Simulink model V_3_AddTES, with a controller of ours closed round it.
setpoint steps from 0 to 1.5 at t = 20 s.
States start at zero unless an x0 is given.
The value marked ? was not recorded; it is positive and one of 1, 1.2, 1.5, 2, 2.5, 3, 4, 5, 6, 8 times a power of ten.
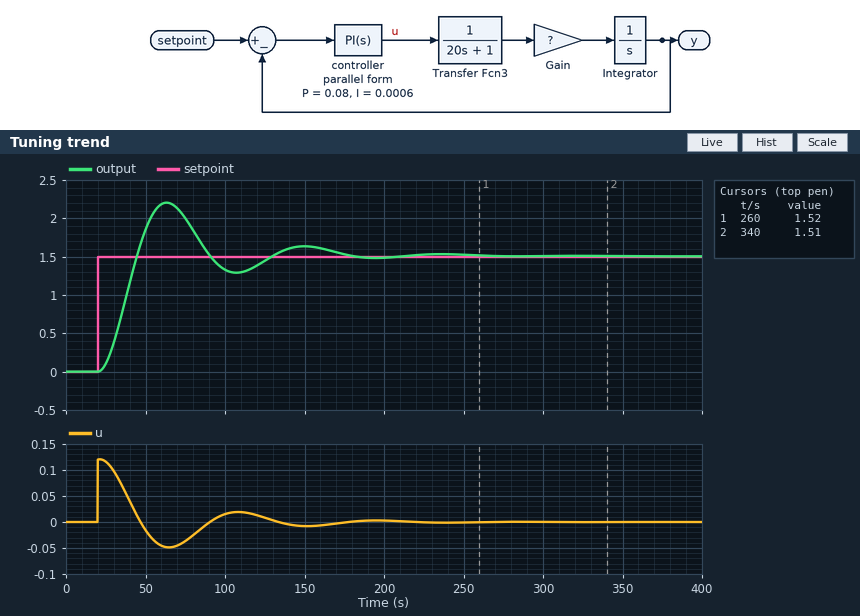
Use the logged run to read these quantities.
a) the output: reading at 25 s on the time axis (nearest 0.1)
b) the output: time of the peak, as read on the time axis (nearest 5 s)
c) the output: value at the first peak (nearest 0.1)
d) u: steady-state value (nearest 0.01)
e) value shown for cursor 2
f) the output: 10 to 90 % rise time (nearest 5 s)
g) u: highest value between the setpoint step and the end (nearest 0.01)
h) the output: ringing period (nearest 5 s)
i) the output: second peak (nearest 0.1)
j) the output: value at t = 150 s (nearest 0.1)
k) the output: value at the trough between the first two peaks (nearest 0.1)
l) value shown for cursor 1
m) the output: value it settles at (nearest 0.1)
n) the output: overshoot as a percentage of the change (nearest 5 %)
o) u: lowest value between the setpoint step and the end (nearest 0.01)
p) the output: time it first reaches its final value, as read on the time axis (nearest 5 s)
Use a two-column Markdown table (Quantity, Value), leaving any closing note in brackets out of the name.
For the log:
| Quantity | Value |
|---|---|
| the output: reading at 25 s on the time axis | 0.1 |
| the output: time of the peak, as read on the time axis | 65 s |
| the output: value at the first peak | 2.2 |
| u: steady-state value | 0.00 |
| value shown for cursor 2 | 1.51 |
| the output: 10 to 90 % rise time | 15 s |
| u: highest value between the setpoint step and the end | 0.12 |
| the output: ringing period | 85 s |
| the output: second peak | 1.6 |
| the output: value at t = 150 s | 1.6 |
| the output: value at the trough between the first two peaks | 1.3 |
| value shown for cursor 1 | 1.52 |
| the output: value it settles at | 1.5 |
| the output: overshoot as a percentage of the change | 45 % |
| u: lowest value between the setpoint step and the end | -0.05 |
| the output: time it first reaches its final value, as read on the time axis | 45 s |
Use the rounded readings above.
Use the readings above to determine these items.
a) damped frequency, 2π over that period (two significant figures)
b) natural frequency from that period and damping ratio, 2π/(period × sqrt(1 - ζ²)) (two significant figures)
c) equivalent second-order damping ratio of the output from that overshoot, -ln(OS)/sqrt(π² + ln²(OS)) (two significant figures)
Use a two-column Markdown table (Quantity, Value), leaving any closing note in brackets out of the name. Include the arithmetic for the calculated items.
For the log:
| Quantity | Value |
|---|---|
| damped frequency, 2π over that period | 2π / 85 = 0.074 rad/s |
| natural frequency from that period and damping ratio, 2π/(period × sqrt(1 - ζ²)) | 2π / (85 × sqrt(1 - 0.25²)) = 0.076 rad/s |
| equivalent second-order damping ratio of the output from that overshoot, -ln(OS)/sqrt(π² + ln²(OS)) | ln(0.45) = -0.799; 0.799 / sqrt(9.870 + 0.638) = 0.25 |
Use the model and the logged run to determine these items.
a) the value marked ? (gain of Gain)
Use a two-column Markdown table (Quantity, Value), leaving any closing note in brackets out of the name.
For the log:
| Quantity | Value |
|---|---|
| the value marked ? | 1.5 |
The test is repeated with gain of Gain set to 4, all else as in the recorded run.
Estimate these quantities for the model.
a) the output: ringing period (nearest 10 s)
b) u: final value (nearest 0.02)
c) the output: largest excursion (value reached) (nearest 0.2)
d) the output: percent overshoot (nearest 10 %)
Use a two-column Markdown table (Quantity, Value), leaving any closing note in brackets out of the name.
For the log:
| Quantity | Value |
|---|---|
| the output: ringing period | 50 s |
| u: final value | 0.00 |
| the output: largest excursion (value reached) | 2.4 |
| the output: percent overshoot | 60 % |
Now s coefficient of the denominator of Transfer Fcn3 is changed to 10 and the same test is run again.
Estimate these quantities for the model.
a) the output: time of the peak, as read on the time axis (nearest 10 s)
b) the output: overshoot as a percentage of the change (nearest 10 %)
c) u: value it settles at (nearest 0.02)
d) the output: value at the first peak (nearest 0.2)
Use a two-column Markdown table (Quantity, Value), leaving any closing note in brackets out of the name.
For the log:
| Quantity | Value |
|---|---|
| the output: time of the peak, as read on the time axis | 50 s |
| the output: overshoot as a percentage of the change | 30 % |
| u: value it settles at | 0.00 |
| the output: value at the first peak | 2.0 |
